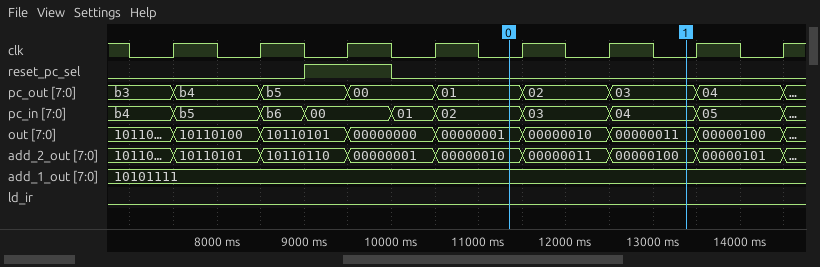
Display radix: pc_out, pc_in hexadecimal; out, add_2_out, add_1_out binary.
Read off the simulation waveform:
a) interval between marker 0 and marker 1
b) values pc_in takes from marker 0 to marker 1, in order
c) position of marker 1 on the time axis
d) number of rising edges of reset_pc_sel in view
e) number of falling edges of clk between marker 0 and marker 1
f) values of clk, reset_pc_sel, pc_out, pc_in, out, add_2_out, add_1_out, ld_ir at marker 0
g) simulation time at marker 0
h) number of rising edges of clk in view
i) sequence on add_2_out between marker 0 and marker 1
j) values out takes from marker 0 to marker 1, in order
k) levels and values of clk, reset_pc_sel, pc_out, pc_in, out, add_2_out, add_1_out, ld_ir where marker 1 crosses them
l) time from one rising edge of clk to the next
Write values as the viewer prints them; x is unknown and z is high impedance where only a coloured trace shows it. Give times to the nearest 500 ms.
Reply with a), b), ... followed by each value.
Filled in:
a) 2000 ms
b) 02, 03, 04
c) 13500 ms
d) 1
e) 2
f) clk=0, reset_pc_sel=0, pc_out=01, pc_in=02, out=00000001, add_2_out=00000010, add_1_out=10101111, ld_ir=0
g) 11500 ms
h) 8
i) 00000010, 00000011, 00000100
j) 00000001, 00000010, 00000011
k) clk=0, reset_pc_sel=0, pc_out=03, pc_in=04, out=00000011, add_2_out=00000100, add_1_out=10101111, ld_ir=0
l) 1000 ms
